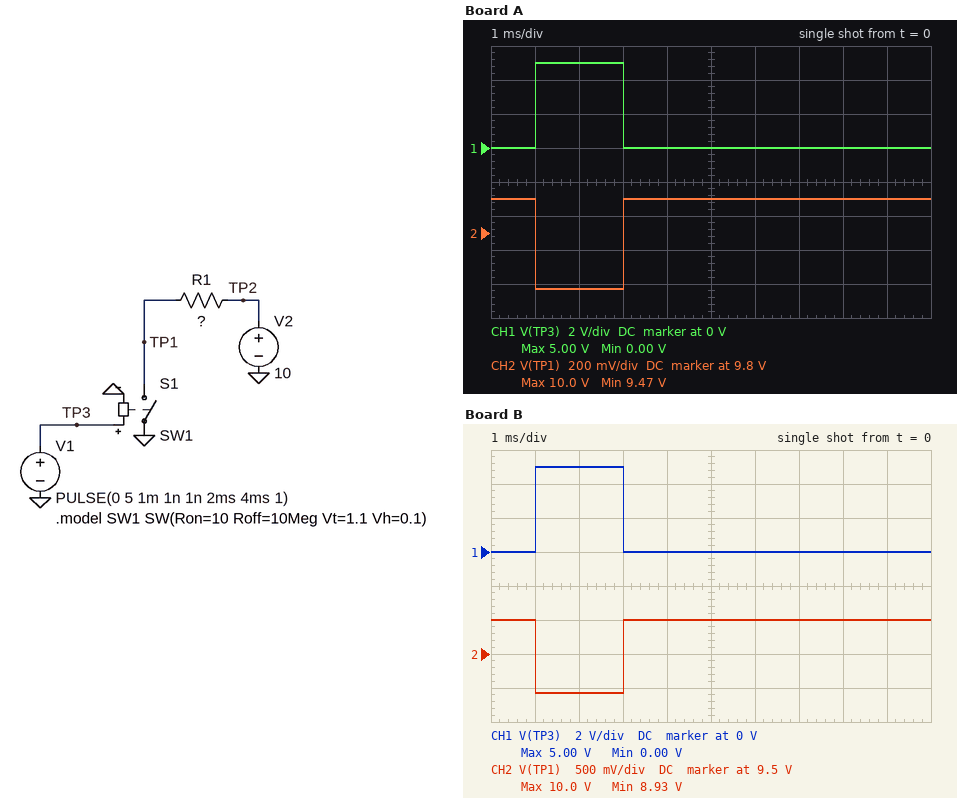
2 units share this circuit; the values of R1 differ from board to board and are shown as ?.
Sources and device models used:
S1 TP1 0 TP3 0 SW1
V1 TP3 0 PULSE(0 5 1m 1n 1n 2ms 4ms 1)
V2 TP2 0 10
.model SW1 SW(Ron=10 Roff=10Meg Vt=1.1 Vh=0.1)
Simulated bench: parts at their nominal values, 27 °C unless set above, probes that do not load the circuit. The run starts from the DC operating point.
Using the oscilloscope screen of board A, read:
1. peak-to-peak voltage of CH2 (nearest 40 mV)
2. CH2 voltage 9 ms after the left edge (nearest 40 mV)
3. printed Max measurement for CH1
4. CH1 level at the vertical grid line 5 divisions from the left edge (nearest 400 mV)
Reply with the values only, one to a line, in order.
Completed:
520 mV
10.00 V
5.00 V
0 V
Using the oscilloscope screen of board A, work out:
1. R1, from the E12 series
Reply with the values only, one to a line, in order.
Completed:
0.56 Ω
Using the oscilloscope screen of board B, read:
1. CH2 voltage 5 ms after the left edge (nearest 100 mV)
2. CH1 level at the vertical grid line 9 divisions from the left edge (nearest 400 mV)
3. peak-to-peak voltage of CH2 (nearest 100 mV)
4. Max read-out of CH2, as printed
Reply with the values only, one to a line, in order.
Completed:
10.0 V
0 V
1.1 V
10.0 V
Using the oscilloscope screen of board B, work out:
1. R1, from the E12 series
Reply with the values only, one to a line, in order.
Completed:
1.2 Ω
